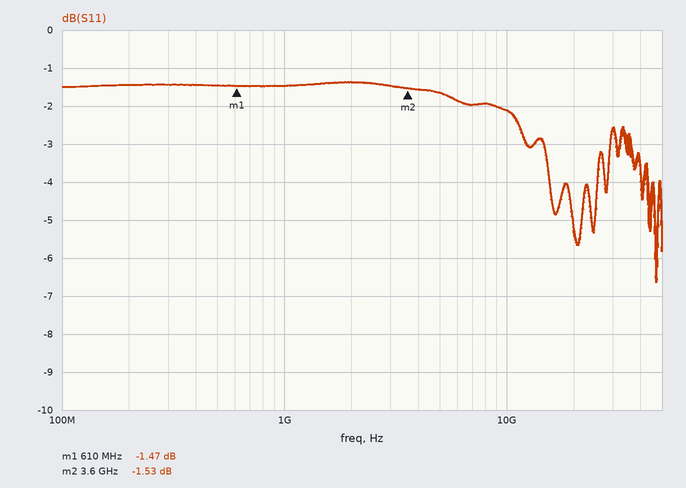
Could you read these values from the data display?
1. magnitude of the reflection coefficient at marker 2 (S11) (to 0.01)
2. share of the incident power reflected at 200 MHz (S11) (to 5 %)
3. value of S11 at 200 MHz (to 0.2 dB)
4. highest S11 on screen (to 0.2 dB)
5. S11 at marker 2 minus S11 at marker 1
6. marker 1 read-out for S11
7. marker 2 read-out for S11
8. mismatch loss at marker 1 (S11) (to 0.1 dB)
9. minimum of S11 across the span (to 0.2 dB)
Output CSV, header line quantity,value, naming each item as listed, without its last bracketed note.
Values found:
quantity,value
magnitude of the reflection coefficient at marker 2 (S11),0.84
share of the incident power reflected at 200 MHz (S11),70 %
value of S11 at 200 MHz,-1.4 dB
highest S11 on screen,-1.4 dB
S11 at marker 2 minus S11 at marker 1,-0.06 dB
marker 1 read-out for S11,-1.47 dB
marker 2 read-out for S11,-1.53 dB
mismatch loss at marker 1 (S11),5.4 dB
minimum of S11 across the span,-6.6 dB
